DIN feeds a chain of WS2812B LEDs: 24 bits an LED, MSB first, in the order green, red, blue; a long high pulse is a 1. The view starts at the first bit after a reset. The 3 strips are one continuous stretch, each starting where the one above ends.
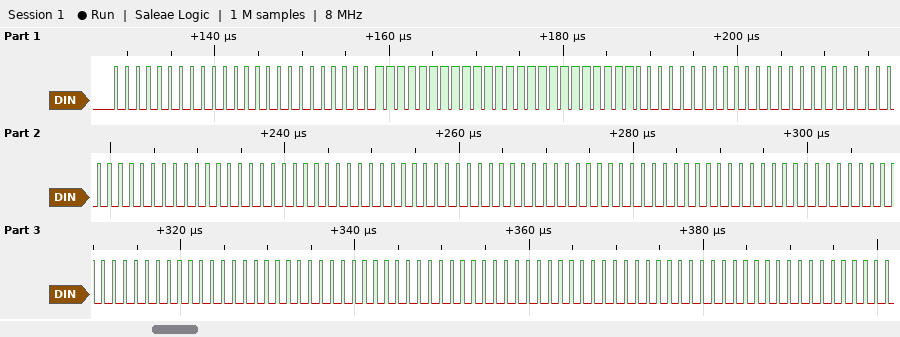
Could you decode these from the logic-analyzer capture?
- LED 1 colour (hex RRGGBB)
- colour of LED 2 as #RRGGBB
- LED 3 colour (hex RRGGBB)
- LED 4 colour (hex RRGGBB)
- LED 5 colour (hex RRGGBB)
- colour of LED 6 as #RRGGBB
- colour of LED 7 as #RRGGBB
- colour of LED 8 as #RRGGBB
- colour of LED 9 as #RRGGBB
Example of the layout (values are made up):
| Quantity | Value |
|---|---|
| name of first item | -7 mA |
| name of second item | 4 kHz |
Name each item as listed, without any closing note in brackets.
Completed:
| Quantity | Value |
|---|---|
| LED 1 colour | #000000 |
| colour of LED 2 as #RRGGBB | #FFFFFF |
| LED 3 colour | #000000 |
| LED 4 colour | #000000 |
| LED 5 colour | #000000 |
| colour of LED 6 as #RRGGBB | #000000 |
| colour of LED 7 as #RRGGBB | #000000 |
| colour of LED 8 as #RRGGBB | #000000 |
| colour of LED 9 as #RRGGBB | #000000 |
